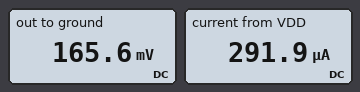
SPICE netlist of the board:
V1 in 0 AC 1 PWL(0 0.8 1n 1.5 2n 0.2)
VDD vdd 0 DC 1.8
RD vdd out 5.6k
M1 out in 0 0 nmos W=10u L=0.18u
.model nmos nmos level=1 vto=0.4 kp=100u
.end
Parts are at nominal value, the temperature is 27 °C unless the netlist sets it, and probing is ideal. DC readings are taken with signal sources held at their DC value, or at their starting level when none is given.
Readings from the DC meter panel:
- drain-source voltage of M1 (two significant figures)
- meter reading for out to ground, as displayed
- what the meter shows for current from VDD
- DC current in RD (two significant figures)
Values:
170 mV
165.6 mV
291.9 µA
290 µA
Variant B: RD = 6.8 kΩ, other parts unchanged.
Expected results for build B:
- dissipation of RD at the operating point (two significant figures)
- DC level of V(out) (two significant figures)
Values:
410 µW
130 mV
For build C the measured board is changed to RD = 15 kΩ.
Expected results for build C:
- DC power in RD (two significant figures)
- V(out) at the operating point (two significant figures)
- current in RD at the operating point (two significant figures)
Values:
200 µW
56 mV
120 µA
